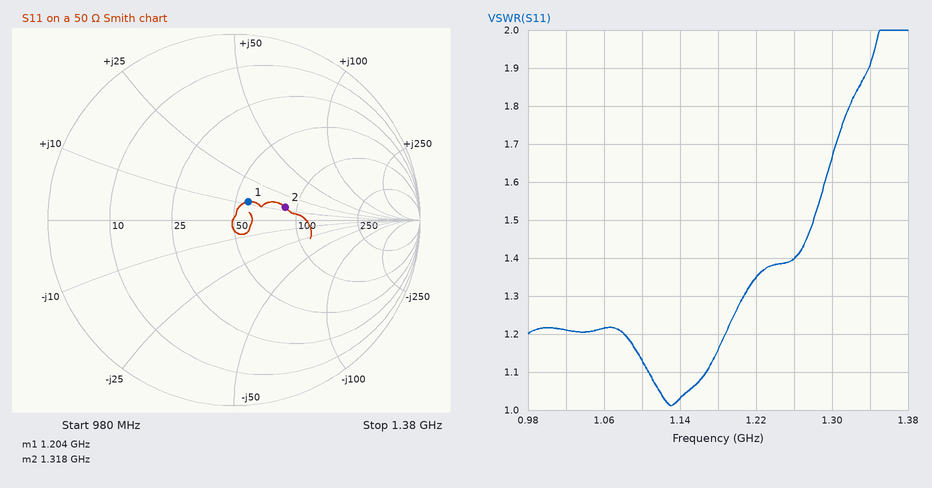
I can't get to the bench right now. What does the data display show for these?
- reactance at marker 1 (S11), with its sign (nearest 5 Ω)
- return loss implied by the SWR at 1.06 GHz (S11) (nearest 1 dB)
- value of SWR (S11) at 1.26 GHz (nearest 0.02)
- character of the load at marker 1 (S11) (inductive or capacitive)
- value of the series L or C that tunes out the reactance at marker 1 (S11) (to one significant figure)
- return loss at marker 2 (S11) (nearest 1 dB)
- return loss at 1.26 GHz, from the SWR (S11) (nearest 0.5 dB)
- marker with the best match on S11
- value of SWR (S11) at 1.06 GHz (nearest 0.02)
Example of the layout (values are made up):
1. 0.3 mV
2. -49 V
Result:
1. +10 Ω
2. 20 dB
3. 1.40
4. inductive
5. 10 pF
6. 11 dB
7. 15.5 dB
8. marker 1
9. 1.22
